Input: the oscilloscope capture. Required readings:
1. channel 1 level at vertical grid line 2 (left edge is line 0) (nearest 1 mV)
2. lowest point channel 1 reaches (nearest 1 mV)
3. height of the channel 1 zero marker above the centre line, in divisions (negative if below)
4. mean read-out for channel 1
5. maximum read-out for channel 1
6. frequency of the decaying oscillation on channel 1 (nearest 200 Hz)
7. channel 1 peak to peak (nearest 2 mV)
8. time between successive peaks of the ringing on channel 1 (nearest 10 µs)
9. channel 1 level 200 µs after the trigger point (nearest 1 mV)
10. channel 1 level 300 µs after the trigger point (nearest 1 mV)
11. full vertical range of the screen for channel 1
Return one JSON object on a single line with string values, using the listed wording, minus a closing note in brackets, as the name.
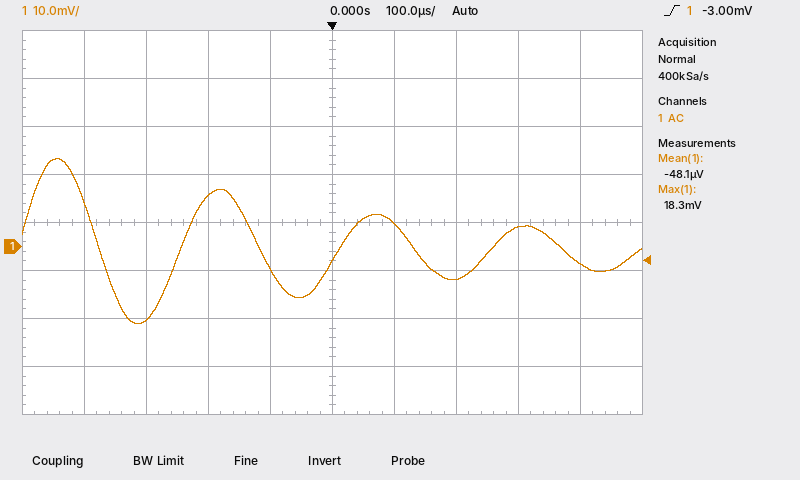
{"channel 1 level at vertical grid line 2 (left edge is line 0)": "-15 mV", "lowest point channel 1 reaches": "-16 mV", "height of the channel 1 zero marker above the centre line, in divisions": "-0.5 div", "mean read-out for channel 1": "-48.1 µV", "maximum read-out for channel 1": "18.3 mV", "frequency of the decaying oscillation on channel 1": "4.0 kHz", "channel 1 peak to peak": "34 mV", "time between successive peaks of the ringing on channel 1": "250 µs", "channel 1 level 200 µs after the trigger point": "-7 mV", "channel 1 level 300 µs after the trigger point": "4 mV", "full vertical range of the screen for channel 1": "80 mV"}
